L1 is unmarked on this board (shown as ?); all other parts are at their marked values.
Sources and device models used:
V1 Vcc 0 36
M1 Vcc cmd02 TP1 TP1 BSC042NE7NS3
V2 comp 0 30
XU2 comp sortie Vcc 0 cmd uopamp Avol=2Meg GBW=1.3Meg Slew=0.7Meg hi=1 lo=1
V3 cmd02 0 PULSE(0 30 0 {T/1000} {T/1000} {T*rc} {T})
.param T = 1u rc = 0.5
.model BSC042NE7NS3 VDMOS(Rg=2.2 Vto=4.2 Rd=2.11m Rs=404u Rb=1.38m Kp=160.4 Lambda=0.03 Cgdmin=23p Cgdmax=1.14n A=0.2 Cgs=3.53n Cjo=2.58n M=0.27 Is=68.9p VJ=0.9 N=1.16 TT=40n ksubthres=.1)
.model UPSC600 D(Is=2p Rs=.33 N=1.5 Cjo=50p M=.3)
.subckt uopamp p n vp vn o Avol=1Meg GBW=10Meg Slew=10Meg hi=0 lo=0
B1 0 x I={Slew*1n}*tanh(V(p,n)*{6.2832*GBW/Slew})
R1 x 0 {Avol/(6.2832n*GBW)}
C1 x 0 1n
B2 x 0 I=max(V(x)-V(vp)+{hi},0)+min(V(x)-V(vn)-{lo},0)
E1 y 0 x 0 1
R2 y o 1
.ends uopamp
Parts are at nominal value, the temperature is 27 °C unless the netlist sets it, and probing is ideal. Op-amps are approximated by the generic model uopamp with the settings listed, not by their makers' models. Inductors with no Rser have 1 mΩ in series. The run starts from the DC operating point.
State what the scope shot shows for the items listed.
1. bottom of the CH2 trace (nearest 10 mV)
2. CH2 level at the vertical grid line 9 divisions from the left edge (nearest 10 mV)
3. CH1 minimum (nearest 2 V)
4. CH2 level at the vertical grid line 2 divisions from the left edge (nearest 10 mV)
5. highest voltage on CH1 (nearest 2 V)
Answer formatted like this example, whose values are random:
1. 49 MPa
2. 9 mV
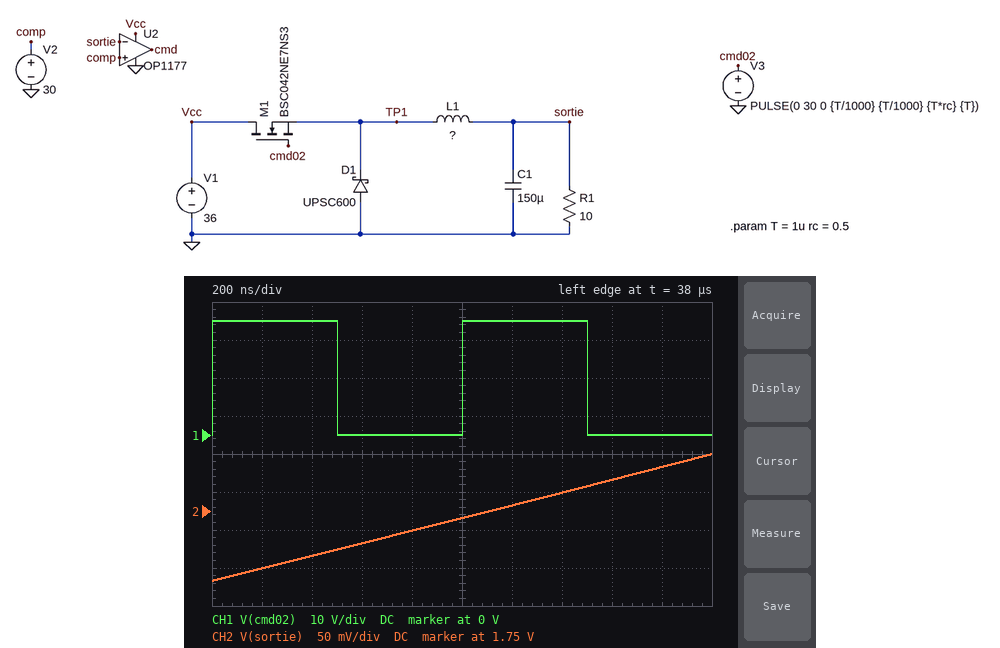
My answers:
1. 1.66 V
2. 1.81 V
3. 0 V
4. 1.69 V
5. 30 V
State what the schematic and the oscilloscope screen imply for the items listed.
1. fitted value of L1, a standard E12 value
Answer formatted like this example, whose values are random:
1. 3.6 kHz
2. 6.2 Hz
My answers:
1. 33 µH
